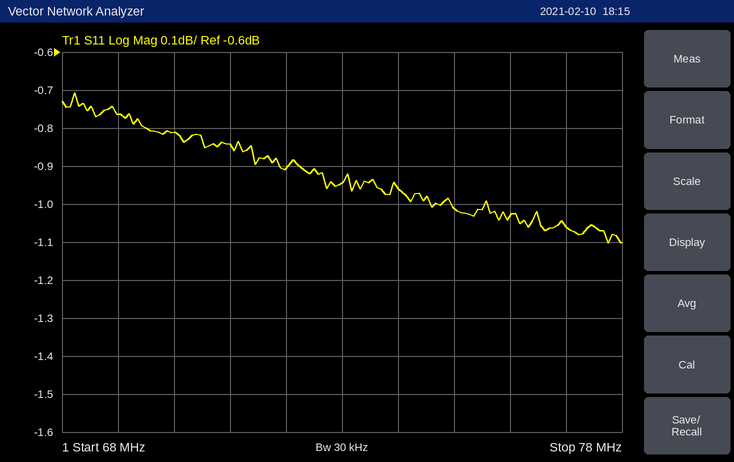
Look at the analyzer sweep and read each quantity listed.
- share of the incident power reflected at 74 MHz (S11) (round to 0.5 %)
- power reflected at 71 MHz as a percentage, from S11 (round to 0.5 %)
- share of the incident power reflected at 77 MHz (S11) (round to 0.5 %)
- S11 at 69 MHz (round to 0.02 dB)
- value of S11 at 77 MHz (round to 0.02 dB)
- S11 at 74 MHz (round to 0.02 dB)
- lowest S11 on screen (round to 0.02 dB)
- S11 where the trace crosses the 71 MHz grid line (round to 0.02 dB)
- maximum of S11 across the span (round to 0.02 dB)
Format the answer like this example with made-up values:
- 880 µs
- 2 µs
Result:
- 80.0 %
- 82.5 %
- 78.5 %
- -0.76 dB
- -1.06 dB
- -0.96 dB
- -1.10 dB
- -0.84 dB
- -0.70 dB
